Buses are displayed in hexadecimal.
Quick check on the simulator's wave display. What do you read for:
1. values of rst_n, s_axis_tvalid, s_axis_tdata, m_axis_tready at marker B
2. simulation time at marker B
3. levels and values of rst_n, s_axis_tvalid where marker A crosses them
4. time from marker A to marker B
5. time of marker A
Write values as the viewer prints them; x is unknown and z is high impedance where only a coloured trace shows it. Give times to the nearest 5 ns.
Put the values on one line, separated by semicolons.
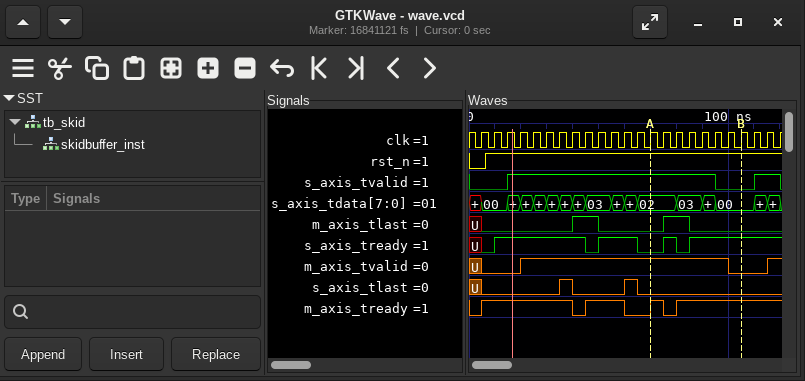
rst_n=1, s_axis_tvalid=0, s_axis_tdata=00, m_axis_tready=1; 105 ns; rst_n=1, s_axis_tvalid=1; 35 ns; 70 ns
